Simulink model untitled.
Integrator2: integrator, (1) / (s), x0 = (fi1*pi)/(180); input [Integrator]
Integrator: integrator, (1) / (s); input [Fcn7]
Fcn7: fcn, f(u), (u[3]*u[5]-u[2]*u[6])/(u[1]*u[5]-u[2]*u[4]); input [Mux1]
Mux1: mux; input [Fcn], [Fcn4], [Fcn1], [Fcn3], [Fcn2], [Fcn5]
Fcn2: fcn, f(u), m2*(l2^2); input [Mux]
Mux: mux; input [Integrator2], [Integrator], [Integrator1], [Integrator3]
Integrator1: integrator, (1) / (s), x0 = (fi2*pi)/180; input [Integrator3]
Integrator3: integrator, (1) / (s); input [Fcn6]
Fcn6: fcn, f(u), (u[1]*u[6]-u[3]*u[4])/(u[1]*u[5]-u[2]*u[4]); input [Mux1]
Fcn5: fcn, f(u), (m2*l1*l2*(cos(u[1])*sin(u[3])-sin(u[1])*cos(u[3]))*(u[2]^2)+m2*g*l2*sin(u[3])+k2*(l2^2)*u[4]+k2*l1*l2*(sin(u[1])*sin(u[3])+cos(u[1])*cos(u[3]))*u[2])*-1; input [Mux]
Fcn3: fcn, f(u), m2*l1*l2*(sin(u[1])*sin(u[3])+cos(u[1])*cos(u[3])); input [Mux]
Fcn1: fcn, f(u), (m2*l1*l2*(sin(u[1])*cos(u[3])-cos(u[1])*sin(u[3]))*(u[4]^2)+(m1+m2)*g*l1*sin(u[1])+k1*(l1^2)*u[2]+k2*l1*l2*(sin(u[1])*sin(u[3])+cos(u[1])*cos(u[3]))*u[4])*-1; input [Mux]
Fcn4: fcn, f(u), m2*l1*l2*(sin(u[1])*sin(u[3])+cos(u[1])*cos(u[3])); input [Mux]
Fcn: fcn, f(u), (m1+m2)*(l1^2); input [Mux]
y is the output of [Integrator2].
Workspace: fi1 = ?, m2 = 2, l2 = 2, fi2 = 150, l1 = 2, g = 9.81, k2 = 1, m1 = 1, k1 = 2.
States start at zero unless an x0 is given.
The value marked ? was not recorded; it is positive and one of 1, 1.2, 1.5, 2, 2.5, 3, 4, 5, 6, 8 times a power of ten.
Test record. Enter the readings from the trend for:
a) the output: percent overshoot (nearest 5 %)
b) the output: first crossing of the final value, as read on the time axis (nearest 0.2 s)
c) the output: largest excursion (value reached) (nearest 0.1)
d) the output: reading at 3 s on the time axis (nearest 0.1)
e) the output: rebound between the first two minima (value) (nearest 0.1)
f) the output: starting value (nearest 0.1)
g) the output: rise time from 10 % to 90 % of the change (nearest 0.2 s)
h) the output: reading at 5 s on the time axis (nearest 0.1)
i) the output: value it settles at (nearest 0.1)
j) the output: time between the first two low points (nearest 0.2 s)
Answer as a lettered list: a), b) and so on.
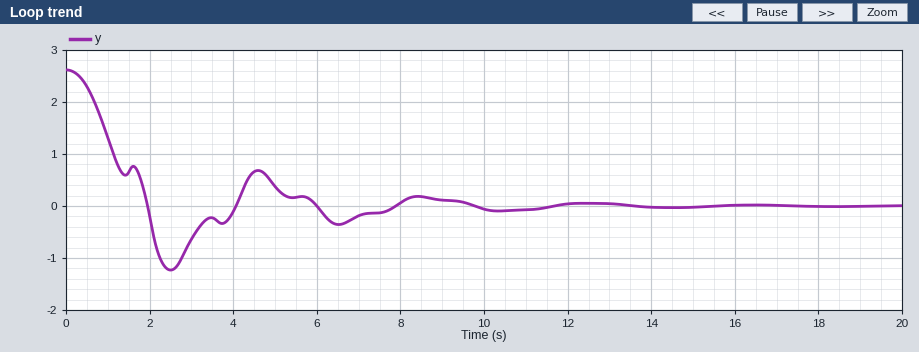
a) 45 %
b) 2.0 s
c) -1.2
d) -0.6
e) 0.7
f) 2.6
g) 1.4 s
h) 0.4
i) 0.0
j) 4.0 s
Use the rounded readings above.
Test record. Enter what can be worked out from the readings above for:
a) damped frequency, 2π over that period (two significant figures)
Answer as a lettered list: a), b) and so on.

a) 1.6 rad/s
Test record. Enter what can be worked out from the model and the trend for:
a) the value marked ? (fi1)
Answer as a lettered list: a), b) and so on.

a) 150
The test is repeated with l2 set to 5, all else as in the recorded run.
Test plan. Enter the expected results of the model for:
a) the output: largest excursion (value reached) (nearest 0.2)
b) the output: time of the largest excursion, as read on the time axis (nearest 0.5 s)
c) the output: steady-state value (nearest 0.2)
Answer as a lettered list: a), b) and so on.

a) -1.4
b) 3.5 s
c) 0.0
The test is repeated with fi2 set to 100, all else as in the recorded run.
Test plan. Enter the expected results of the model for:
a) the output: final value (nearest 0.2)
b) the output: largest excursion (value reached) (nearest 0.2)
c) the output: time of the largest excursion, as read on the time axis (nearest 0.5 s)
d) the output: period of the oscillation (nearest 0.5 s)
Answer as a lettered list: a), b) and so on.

a) 0.0
b) -0.8
c) 3.0 s
d) 3.5 s
